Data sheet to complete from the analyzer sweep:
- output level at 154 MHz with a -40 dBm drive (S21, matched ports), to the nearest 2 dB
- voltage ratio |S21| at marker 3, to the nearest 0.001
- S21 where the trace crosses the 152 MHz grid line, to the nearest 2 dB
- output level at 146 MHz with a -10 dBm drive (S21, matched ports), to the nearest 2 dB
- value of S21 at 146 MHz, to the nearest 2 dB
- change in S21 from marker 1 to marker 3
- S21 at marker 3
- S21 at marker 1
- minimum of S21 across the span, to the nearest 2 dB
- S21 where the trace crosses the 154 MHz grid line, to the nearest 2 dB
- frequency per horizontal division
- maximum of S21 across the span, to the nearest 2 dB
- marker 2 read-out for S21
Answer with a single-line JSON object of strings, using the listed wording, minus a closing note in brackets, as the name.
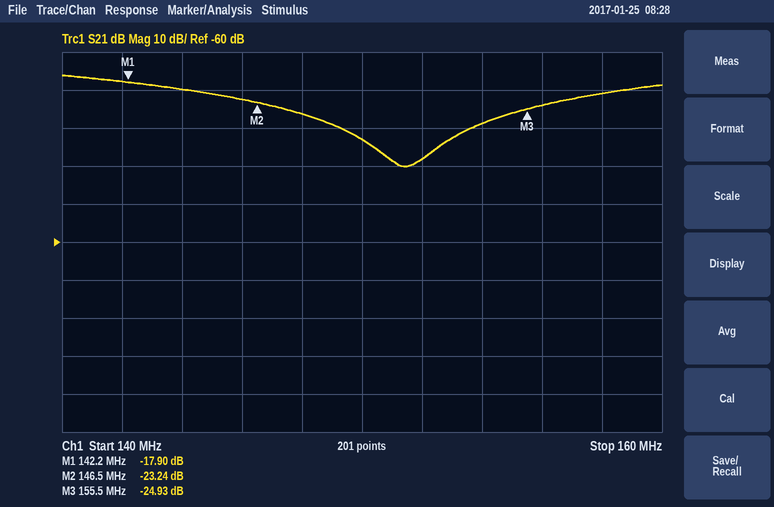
{"output level at 154 MHz with a -40 dBm drive (S21, matched ports), to the nearest 2 dB": "-68 dBm", "voltage ratio |S21| at marker 3, to the nearest 0.001": "0.057", "S21 where the trace crosses the 152 MHz grid line, to the nearest 2 dB": "-38 dB", "output level at 146 MHz with a -10 dBm drive (S21, matched ports), to the nearest 2 dB": "-32 dBm", "value of S21 at 146 MHz, to the nearest 2 dB": "-22 dB", "change in S21 from marker 1 to marker 3": "-7.03 dB", "S21 at marker 3": "-24.93 dB", "S21 at marker 1": "-17.90 dB", "minimum of S21 across the span, to the nearest 2 dB": "-40 dB", "S21 where the trace crosses the 154 MHz grid line, to the nearest 2 dB": "-28 dB", "frequency per horizontal division": "2 MHz", "maximum of S21 across the span, to the nearest 2 dB": "-16 dB", "marker 2 read-out for S21": "-23.24 dB"}
